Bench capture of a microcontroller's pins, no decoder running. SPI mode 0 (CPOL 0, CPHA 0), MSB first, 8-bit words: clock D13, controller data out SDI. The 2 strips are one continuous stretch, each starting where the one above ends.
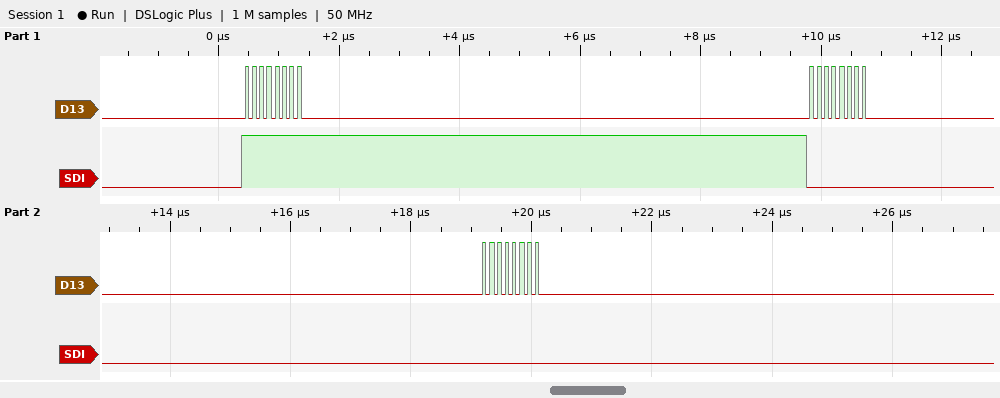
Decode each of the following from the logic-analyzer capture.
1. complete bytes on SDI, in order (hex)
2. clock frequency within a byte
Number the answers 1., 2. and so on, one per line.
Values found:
1. FF 00 00
2. 8 MHz
